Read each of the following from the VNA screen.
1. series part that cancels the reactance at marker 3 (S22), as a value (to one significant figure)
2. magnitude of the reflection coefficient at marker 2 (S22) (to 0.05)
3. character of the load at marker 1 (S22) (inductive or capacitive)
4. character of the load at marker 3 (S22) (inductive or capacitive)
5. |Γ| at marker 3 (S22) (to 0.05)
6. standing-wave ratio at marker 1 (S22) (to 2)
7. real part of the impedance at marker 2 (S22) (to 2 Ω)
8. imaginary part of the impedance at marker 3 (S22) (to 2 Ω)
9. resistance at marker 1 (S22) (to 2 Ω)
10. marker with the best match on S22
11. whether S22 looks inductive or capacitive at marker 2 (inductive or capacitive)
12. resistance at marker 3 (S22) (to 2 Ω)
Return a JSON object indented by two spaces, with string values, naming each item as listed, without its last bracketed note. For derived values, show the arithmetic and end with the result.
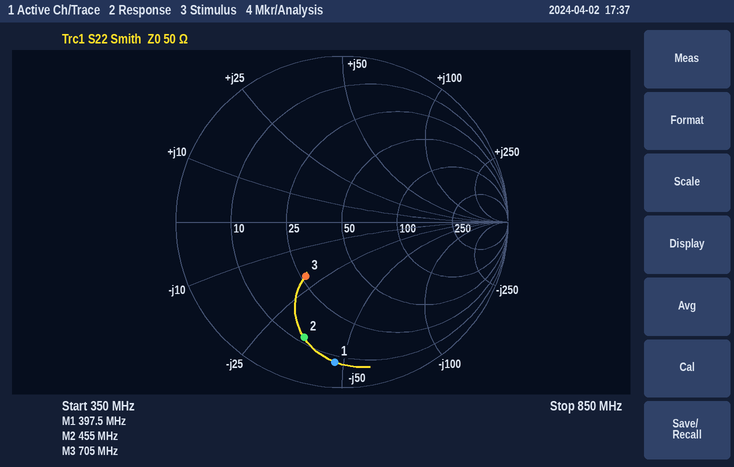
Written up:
{
  "series part that cancels the reactance at marker 3 (S22), as a value": "L = 20 Ω/(2π × 705 MHz) ≈ 5 nH",
  "magnitude of the reflection coefficient at marker 2 (S22)": "0.75",
  "character of the load at marker 1 (S22)": "capacitive",
  "character of the load at marker 3 (S22)": "capacitive",
  "|Γ| at marker 3 (S22)": "0.40",
  "standing-wave ratio at marker 1 (S22)": "12",
  "real part of the impedance at marker 2 (S22)": "12 Ω",
  "imaginary part of the impedance at marker 3 (S22)": "-20 Ω",
  "resistance at marker 1 (S22)": "8 Ω",
  "marker with the best match on S22": "marker 3",
  "whether S22 looks inductive or capacitive at marker 2": "capacitive",
  "resistance at marker 3 (S22)": "26 Ω"
}
